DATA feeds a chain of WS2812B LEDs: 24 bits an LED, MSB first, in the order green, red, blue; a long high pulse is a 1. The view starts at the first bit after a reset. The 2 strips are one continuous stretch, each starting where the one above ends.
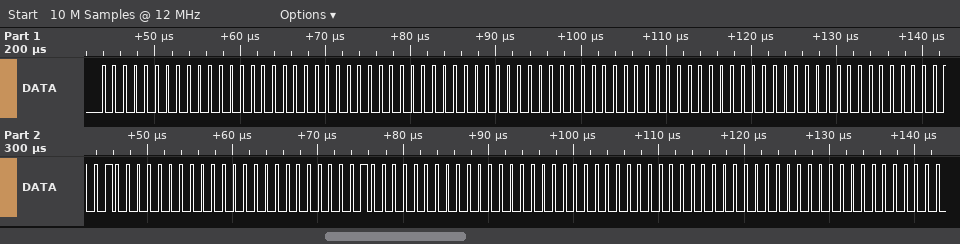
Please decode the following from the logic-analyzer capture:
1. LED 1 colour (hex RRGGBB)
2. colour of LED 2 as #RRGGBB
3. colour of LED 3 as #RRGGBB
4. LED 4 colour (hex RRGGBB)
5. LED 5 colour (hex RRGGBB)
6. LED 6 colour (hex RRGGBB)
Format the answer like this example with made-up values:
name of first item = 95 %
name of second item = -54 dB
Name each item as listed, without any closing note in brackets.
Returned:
LED 1 colour = #000000
colour of LED 2 as #RRGGBB = #000000
colour of LED 3 as #RRGGBB = #000000
LED 4 colour = #400000
LED 5 colour = #400000
LED 6 colour = #000000
